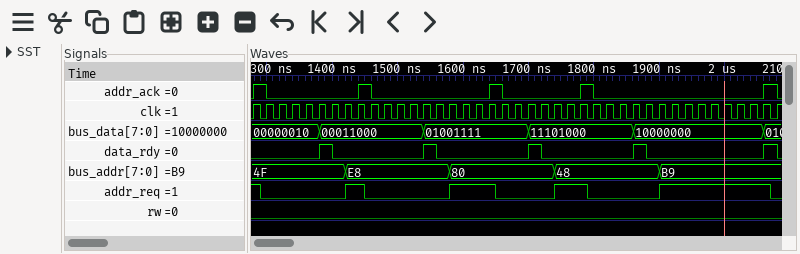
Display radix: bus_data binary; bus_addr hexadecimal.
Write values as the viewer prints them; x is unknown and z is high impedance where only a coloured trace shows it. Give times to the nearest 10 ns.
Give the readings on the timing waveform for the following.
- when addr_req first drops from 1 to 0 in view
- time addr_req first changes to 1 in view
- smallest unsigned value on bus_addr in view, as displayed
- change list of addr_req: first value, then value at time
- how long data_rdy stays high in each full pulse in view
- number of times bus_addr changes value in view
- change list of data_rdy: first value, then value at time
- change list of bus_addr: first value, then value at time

1290 ns
1420 ns
48
1, 0 at 1290 ns, 1 at 1420 ns, 0 at 1450 ns, 1 at 1580 ns, 0 at 1650 ns, 1 at 1740 ns, 0 at 1790 ns, 1 at 1900 ns, 0 at 2070 ns
20 ns, 20 ns, 20 ns, 20 ns, 20 ns
4
0, 1 at 1380 ns, 0 at 1400 ns, 1 at 1540 ns, 0 at 1560 ns, 1 at 1700 ns, 0 at 1720 ns, 1 at 1860 ns, 0 at 1880 ns, 1 at 2060 ns, 0 at 2080 ns
4F, E8 at 1420 ns, 80 at 1580 ns, 48 at 1740 ns, B9 at 1900 ns
